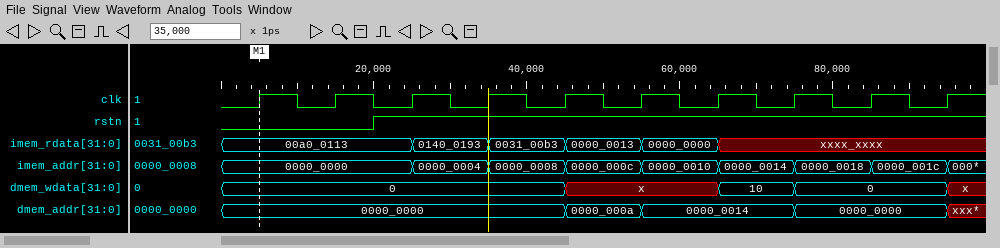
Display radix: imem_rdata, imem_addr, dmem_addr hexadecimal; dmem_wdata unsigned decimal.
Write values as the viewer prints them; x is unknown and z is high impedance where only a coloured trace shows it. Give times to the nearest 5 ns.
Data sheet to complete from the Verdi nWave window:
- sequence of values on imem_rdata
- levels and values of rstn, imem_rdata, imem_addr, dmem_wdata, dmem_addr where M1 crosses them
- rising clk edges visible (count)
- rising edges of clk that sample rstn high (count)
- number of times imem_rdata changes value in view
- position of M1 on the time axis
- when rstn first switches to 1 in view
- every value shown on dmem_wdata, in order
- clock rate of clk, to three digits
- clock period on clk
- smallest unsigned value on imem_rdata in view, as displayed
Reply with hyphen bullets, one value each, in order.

- 00a0_0113, 0140_0193, 0031_00b3, 0000_0013, 0000_0000, xxxx_xxxx
- rstn=0, imem_rdata=00a0_0113, imem_addr=0000_0000, dmem_wdata=0, dmem_addr=0000_0000
- 10
- 8
- 5
- 5 ns
- 20 ns
- 0, x, 10, 0, x
- 100 MHz
- 10 ns
- 0000_0000
